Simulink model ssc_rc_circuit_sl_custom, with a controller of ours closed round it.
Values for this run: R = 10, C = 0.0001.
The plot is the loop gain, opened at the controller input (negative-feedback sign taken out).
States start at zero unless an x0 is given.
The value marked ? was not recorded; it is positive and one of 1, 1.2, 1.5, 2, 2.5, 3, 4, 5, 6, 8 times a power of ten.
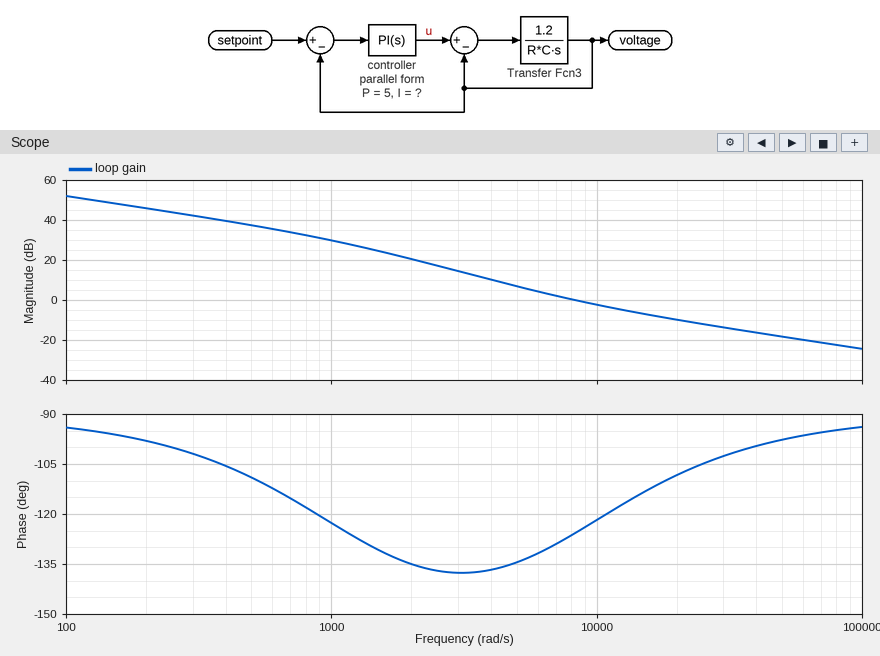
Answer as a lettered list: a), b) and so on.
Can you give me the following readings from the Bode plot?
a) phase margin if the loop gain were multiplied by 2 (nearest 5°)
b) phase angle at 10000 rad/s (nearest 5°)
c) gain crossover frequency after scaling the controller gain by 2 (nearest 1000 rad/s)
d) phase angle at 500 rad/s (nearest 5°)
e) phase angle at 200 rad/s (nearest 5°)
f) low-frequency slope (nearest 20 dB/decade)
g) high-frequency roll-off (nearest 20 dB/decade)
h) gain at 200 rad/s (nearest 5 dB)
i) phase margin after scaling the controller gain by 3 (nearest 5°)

a) 65°
b) -120°
c) 14000 rad/s
d) -110°
e) -100°
f) -20 dB/decade
g) -20 dB/decade
h) 45 dB
i) 70°
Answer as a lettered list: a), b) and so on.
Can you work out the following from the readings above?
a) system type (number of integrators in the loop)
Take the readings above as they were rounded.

a) 1
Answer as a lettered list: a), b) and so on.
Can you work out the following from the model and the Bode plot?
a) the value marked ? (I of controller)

a) 40000
